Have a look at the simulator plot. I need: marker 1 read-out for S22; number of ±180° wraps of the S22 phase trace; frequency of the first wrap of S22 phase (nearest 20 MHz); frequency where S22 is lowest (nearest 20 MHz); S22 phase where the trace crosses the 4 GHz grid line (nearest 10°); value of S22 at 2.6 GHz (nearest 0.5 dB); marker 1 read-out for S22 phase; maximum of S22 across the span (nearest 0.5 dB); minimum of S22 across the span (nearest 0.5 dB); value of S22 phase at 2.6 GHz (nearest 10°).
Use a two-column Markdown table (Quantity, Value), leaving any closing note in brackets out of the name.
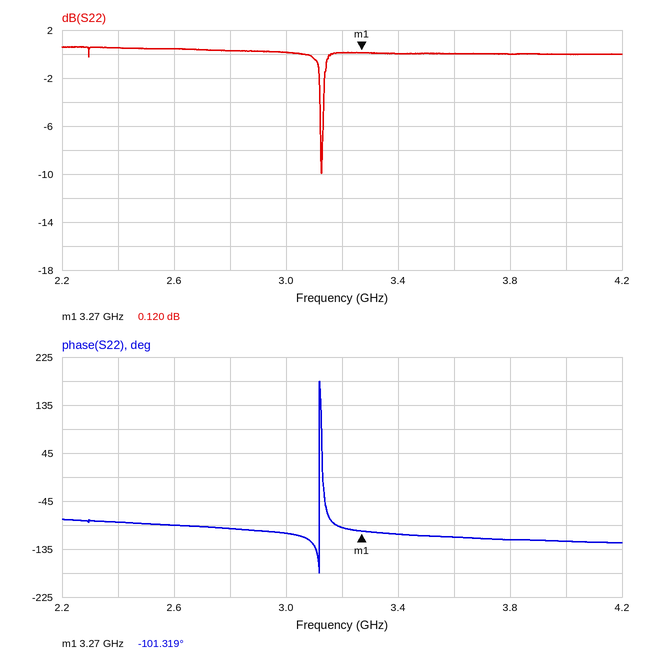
| Quantity | Value |
|---|---|
| marker 1 read-out for S22 | 0.120 dB |
| number of ±180° wraps of the S22 phase trace | 1 |
| frequency of the first wrap of S22 phase | 3.12 GHz |
| frequency where S22 is lowest | 3.12 GHz |
| S22 phase where the trace crosses the 4 GHz grid line | -120° |
| value of S22 at 2.6 GHz | 0.5 dB |
| marker 1 read-out for S22 phase | -101.319° |
| maximum of S22 across the span | 0.5 dB |
| minimum of S22 across the span | -10.0 dB |
| value of S22 phase at 2.6 GHz | -90° |
